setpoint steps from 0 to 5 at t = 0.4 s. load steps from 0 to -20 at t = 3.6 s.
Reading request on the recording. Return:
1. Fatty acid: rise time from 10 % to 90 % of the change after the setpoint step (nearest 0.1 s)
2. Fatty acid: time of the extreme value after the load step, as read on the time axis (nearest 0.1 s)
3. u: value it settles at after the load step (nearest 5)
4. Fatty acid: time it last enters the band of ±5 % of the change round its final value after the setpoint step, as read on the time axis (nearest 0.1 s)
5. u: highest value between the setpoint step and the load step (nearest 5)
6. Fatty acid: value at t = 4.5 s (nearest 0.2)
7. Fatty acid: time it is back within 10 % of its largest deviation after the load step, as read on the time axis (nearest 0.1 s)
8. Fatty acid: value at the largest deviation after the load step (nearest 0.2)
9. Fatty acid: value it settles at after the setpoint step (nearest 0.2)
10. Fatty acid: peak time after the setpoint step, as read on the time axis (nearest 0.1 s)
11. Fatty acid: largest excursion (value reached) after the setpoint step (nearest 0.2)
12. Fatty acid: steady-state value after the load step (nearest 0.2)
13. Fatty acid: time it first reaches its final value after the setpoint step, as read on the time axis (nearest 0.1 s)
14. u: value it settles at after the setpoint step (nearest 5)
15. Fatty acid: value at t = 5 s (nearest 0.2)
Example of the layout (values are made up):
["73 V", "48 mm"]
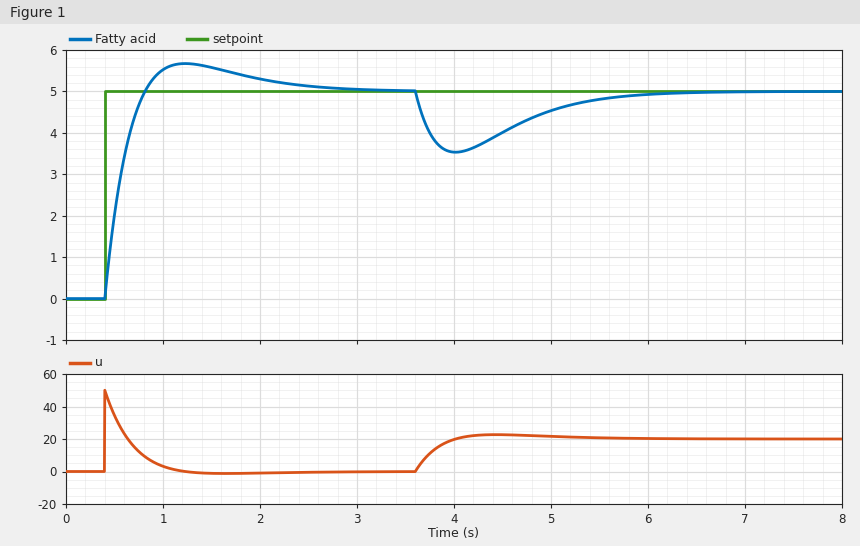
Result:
["0.3 s", "4.0 s", "20", "2.1 s", "50", "4.0", "5.6 s", "3.6", "5.0", "1.2 s", "5.6", "5.0", "0.8 s", "0", "4.6"]
